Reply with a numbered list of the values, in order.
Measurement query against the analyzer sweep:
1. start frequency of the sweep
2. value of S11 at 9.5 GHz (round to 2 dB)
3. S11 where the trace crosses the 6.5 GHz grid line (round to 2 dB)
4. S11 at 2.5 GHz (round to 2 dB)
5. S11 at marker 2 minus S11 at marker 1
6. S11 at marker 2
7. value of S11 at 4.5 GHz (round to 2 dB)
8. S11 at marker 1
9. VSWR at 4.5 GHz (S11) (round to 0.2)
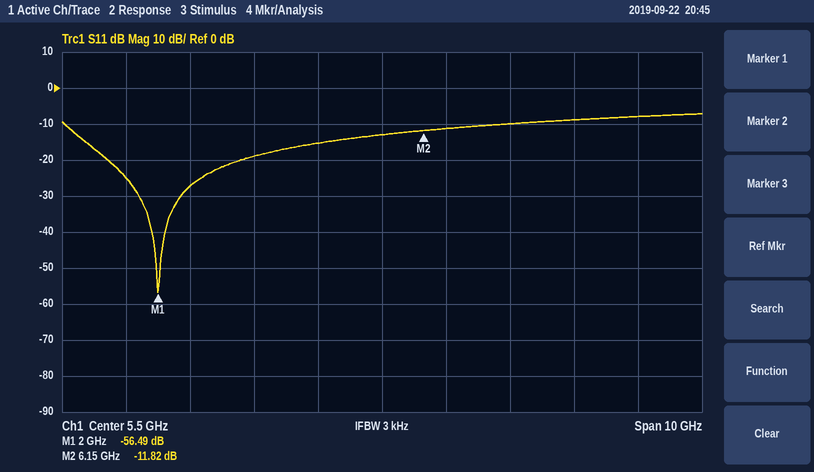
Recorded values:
1. 500 MHz
2. -8 dB
3. -12 dB
4. -28 dB
5. 44.67 dB
6. -11.82 dB
7. -16 dB
8. -56.49 dB
9. 1.4
